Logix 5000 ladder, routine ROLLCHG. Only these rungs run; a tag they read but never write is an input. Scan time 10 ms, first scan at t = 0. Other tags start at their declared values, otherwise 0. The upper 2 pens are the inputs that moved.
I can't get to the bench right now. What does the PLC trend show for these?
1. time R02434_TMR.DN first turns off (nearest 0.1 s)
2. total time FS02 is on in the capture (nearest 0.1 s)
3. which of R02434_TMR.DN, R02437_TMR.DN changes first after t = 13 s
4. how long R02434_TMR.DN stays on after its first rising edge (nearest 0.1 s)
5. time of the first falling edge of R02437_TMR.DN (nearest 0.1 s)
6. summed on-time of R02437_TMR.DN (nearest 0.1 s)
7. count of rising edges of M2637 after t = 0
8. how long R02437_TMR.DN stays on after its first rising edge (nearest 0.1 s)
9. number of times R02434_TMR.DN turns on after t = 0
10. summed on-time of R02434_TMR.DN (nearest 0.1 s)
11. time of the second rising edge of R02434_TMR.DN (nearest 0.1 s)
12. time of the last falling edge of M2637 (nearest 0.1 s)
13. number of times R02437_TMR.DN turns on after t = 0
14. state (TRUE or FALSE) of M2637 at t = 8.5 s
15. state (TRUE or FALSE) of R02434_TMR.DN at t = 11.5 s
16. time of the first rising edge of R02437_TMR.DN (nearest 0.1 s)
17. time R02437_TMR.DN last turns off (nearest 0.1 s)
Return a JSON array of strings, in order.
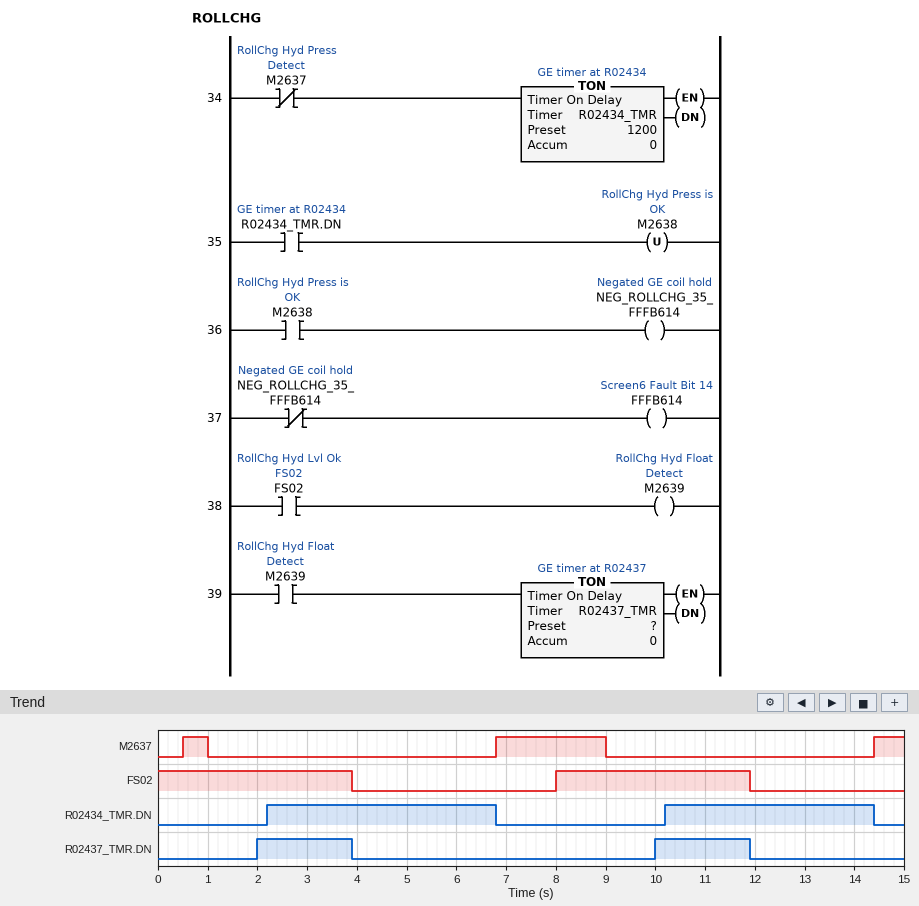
["6.8 s", "7.8 s", "R02434_TMR.DN", "4.6 s", "3.9 s", "3.8 s", "3", "1.9 s", "2", "8.8 s", "10.2 s", "9.0 s", "2", "TRUE", "TRUE", "2.0 s", "11.9 s"]
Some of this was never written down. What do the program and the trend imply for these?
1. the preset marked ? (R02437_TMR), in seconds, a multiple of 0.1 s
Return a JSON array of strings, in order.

["2.0 s"]
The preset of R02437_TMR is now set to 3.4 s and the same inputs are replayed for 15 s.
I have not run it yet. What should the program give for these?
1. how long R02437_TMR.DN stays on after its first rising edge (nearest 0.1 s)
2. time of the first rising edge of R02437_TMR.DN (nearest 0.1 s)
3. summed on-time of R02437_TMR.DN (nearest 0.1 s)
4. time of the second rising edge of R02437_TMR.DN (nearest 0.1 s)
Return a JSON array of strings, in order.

["0.5 s", "3.4 s", "1.0 s", "11.4 s"]
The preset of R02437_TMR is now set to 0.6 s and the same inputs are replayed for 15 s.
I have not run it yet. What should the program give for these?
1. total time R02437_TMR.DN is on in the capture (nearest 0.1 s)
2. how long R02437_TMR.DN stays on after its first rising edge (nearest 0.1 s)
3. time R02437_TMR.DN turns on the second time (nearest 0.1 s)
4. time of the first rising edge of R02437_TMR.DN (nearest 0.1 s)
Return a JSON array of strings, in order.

["6.6 s", "3.3 s", "8.6 s", "0.6 s"]
